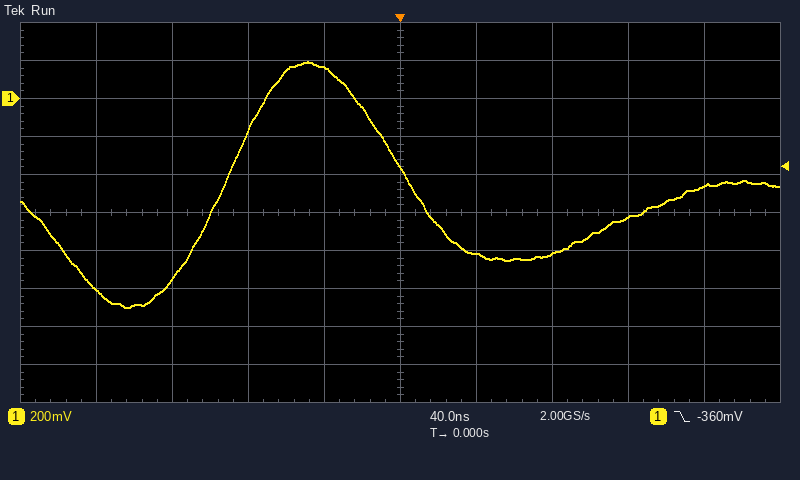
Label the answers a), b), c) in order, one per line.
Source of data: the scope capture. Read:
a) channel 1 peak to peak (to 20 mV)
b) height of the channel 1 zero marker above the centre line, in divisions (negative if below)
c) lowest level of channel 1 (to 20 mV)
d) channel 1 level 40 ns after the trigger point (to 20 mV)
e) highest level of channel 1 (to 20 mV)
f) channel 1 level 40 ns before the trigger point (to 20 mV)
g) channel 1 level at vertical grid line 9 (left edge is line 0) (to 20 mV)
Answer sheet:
a) 1.30 V
b) +3.0 div
c) -1.10 V
d) -820 mV
e) 200 mV
f) 160 mV
g) -460 mV
